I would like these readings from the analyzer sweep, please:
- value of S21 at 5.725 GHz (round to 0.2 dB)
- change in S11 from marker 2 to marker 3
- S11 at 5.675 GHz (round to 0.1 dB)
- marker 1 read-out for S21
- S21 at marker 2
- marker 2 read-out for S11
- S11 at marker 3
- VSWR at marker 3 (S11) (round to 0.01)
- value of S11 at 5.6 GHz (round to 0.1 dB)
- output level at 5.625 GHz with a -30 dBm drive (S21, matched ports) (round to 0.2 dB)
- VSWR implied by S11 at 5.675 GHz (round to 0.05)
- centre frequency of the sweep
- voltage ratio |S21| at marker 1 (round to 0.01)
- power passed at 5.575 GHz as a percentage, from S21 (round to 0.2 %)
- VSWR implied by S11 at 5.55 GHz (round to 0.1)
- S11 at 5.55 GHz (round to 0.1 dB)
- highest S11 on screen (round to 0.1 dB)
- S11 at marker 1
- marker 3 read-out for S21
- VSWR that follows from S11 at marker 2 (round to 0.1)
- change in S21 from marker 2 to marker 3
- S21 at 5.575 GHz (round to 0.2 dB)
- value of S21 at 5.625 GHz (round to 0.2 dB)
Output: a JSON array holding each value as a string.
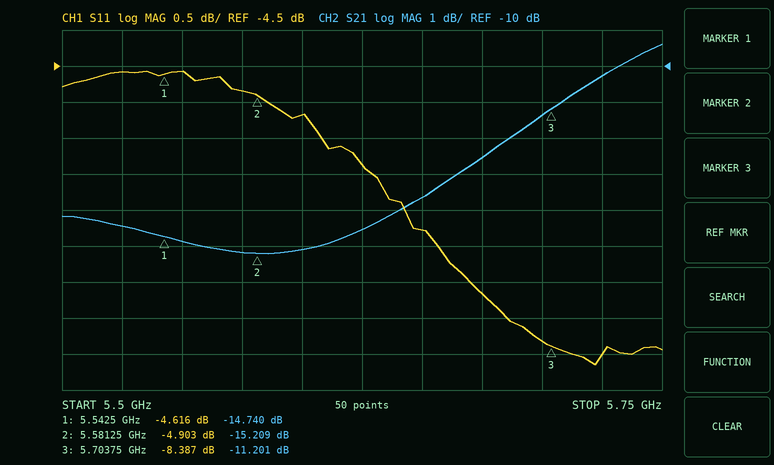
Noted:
["-10.2 dB", "-3.484 dB", "-7.7 dB", "-14.740 dB", "-15.209 dB", "-4.903 dB", "-8.387 dB", "2.23", "-5.2 dB", "-44.6 dBm", "2.40", "5.625 GHz", "0.18", "3.0 %", "3.9", "-4.6 dB", "-4.6 dB", "-4.616 dB", "-11.201 dB", "3.6", "4.008 dB", "-15.2 dB", "-14.6 dB"]
